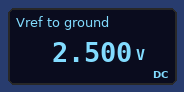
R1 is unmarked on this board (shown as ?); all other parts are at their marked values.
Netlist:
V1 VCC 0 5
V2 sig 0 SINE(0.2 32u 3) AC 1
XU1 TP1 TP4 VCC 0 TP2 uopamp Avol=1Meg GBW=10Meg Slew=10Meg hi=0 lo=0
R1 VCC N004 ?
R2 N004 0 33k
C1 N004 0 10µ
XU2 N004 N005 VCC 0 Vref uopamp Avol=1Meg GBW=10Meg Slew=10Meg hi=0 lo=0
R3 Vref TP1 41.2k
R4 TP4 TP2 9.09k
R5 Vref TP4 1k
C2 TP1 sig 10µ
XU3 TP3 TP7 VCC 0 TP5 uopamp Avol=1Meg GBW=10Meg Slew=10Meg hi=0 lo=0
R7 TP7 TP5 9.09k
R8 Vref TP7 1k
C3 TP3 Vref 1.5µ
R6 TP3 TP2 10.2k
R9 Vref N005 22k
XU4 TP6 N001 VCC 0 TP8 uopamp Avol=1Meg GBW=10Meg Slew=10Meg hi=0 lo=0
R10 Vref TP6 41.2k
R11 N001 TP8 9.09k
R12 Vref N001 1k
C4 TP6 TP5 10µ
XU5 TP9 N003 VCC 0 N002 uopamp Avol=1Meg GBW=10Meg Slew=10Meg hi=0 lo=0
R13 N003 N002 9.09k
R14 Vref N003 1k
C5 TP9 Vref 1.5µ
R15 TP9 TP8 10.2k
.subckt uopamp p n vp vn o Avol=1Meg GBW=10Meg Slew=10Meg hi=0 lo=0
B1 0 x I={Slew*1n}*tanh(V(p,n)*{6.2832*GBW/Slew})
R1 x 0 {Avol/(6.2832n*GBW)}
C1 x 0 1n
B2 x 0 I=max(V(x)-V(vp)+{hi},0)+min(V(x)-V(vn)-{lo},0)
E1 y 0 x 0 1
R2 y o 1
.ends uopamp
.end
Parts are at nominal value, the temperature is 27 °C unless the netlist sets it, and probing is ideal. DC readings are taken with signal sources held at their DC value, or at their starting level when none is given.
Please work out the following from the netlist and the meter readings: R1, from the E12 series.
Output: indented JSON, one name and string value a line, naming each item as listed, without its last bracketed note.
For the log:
{
  "R1, from the E12 series": "33 kΩ"
}
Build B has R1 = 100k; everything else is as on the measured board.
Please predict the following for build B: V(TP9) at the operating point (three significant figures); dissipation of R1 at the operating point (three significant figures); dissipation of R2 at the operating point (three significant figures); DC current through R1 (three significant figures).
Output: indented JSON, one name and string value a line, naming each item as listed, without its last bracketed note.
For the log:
{
  "V(TP9) at the operating point": "1.24 V",
  "dissipation of R1 at the operating point": "141 µW",
  "dissipation of R2 at the operating point": "46.6 µW",
  "DC current through R1": "37.6 µA"
}
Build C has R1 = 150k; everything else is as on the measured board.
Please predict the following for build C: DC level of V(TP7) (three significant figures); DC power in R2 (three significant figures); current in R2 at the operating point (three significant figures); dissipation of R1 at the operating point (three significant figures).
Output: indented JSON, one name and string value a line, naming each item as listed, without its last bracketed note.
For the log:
{
  "DC level of V(TP7)": "902 mV",
  "DC power in R2": "24.6 µW",
  "current in R2 at the operating point": "27.3 µA",
  "dissipation of R1 at the operating point": "112 µW"
}
